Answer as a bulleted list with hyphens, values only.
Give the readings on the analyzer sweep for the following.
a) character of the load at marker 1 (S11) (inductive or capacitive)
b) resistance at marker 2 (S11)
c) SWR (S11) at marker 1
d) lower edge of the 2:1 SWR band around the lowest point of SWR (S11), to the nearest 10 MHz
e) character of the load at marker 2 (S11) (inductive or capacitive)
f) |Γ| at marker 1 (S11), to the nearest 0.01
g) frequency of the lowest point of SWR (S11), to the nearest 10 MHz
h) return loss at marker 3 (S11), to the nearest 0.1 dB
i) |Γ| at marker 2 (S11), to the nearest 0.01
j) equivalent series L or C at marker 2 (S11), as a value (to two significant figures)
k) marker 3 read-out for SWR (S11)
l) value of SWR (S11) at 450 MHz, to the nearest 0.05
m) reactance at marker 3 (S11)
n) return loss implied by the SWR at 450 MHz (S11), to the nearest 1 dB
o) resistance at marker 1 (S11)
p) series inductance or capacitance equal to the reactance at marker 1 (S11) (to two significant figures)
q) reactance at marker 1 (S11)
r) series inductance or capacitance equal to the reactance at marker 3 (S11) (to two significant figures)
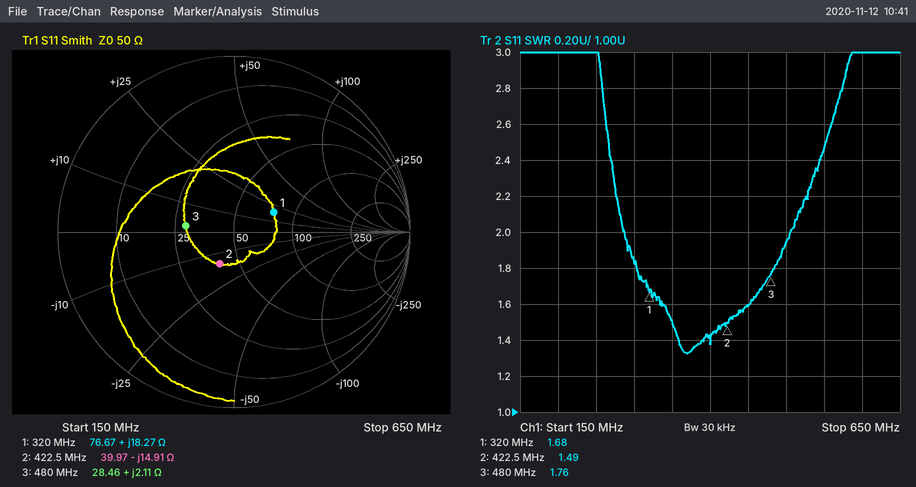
- inductive
- 39.97 Ω
- 1.68
- 290 MHz
- capacitive
- 0.25
- 370 MHz
- 11.2 dB
- 0.20
- 25 pF
- 1.76
- 1.60
- +2.11 Ω
- 13 dB
- 76.67 Ω
- 9.1 nH
- +18.27 Ω
- 700 pH
